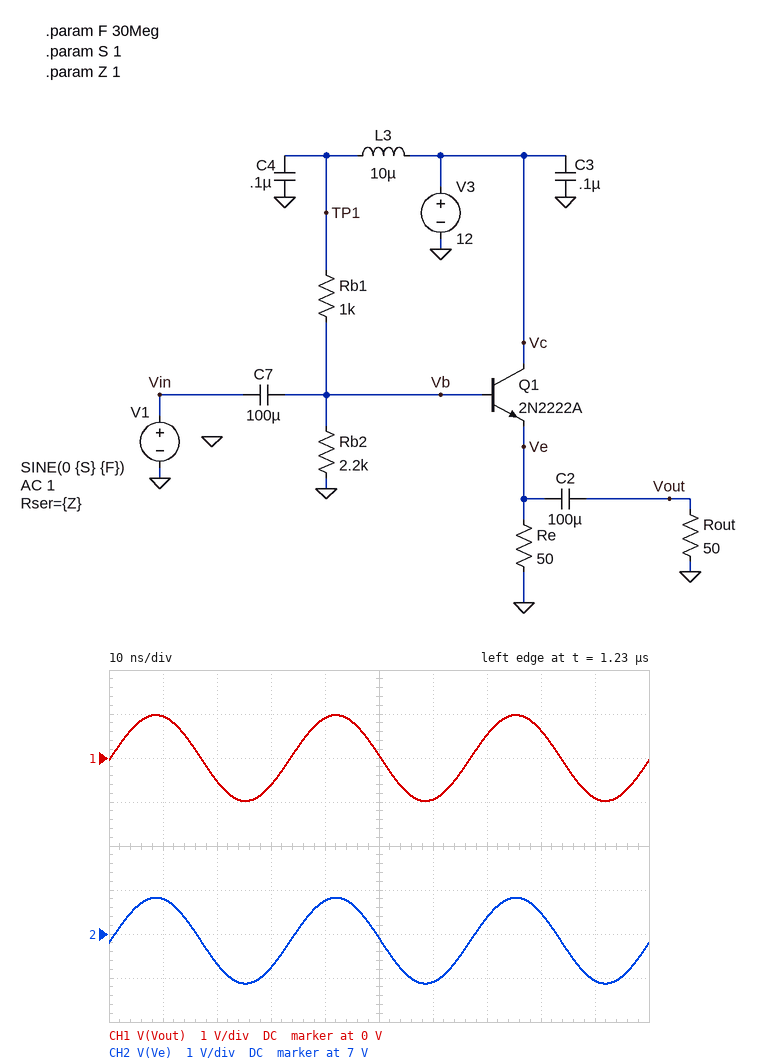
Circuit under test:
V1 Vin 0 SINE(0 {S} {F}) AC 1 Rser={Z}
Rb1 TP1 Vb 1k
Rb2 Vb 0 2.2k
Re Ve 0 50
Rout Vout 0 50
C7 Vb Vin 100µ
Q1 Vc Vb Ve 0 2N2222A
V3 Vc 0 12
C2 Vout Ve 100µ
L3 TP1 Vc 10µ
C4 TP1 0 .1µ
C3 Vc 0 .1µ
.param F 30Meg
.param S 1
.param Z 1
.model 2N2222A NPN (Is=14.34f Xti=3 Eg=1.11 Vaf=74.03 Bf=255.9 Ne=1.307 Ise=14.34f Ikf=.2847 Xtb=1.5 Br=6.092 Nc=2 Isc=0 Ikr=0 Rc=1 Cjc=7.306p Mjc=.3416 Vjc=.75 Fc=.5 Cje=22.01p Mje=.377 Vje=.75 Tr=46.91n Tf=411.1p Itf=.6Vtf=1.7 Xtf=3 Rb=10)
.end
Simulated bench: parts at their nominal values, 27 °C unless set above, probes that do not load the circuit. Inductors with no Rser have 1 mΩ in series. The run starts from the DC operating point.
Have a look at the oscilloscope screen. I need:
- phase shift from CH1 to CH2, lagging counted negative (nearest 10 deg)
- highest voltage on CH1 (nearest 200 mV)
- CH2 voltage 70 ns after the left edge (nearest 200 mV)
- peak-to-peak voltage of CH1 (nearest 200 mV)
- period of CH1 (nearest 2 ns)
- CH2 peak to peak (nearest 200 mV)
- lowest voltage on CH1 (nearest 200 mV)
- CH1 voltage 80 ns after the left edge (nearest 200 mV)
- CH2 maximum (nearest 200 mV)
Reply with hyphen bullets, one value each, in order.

- 0 deg
- 1.0 V
- 7.4 V
- 2.0 V
- 34 ns
- 2.0 V
- -1.0 V
- 600 mV
- 7.8 V
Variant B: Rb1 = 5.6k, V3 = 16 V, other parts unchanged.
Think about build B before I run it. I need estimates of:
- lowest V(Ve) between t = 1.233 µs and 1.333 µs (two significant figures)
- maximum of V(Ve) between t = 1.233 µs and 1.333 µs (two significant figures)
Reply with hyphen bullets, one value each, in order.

- 2.3 V
- 4.2 V
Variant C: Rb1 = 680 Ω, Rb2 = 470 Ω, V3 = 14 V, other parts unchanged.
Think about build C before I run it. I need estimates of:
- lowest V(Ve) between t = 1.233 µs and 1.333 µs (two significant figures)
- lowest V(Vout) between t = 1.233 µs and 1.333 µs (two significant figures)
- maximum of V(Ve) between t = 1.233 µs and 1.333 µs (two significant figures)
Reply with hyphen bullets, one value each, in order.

- 3.8 V
- -970 mV
- 5.8 V
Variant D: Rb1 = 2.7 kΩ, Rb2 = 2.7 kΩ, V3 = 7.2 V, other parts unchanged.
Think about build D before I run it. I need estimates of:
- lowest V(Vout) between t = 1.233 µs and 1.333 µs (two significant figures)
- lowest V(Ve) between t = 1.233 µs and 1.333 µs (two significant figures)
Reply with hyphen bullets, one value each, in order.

- -950 mV
- 1.5 V
